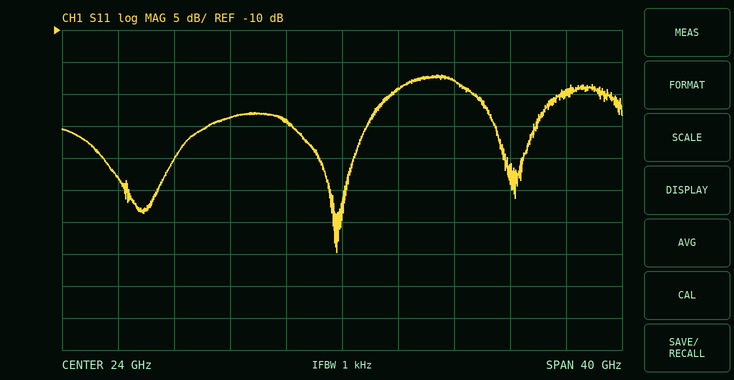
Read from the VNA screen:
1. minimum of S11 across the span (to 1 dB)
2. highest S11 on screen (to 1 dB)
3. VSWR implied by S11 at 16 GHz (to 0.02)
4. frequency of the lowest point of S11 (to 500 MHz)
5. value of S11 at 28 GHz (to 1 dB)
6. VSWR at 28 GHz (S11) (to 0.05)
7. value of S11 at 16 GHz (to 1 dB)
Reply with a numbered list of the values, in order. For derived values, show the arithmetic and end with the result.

1. -45 dB
2. -17 dB
3. |Γ| = 10^(-24/20) = 0.0631; VSWR = (1 + 0.0631)/(1 − 0.0631) ≈ 1.13, so 1.14 to the nearest 0.02
4. 23.5 GHz
5. -19 dB
6. |Γ| = 10^(-19/20) = 0.1122; VSWR = (1 + 0.1122)/(1 − 0.1122) ≈ 1.25
7. -24 dB
